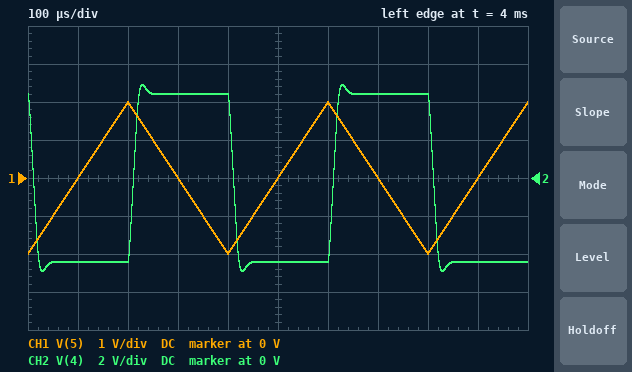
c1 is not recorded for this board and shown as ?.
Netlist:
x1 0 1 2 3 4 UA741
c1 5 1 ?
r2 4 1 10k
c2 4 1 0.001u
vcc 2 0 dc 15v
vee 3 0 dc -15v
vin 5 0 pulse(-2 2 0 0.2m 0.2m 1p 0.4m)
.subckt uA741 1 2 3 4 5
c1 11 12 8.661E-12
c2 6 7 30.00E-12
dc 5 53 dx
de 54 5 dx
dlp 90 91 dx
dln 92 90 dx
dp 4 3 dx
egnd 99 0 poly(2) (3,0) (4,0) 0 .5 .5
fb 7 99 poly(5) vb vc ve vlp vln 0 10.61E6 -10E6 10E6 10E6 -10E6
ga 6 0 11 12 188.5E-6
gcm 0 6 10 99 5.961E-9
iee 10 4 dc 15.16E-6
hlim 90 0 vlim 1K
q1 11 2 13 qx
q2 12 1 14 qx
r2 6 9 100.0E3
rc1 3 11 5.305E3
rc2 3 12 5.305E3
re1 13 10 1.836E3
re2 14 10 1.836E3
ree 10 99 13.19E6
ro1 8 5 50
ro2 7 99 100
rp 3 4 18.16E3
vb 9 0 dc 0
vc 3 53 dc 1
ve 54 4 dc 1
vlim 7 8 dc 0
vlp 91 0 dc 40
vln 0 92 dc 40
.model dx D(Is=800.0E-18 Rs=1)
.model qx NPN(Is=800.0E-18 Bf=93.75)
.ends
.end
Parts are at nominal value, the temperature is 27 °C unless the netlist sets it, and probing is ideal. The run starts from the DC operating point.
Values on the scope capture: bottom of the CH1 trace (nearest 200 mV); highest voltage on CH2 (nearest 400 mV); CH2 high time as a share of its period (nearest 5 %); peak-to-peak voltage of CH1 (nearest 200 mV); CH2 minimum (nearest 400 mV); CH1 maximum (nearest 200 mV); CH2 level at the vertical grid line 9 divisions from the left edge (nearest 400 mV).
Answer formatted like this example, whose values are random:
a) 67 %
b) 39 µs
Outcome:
a) -2.0 V
b) 4.8 V
c) 50 %
d) 4.0 V
e) -4.8 V
f) 2.0 V
g) -4.4 V
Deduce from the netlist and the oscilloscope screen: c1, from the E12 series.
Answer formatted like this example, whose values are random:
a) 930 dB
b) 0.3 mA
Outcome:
a) 22 nF
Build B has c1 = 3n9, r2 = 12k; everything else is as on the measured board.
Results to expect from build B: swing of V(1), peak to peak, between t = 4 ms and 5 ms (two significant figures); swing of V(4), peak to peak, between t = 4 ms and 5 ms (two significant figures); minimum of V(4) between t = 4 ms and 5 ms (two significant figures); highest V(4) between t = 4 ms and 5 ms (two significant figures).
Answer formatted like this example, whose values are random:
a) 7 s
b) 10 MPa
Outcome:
a) 45 mV
b) 1.9 V
c) -940 mV
d) 940 mV
